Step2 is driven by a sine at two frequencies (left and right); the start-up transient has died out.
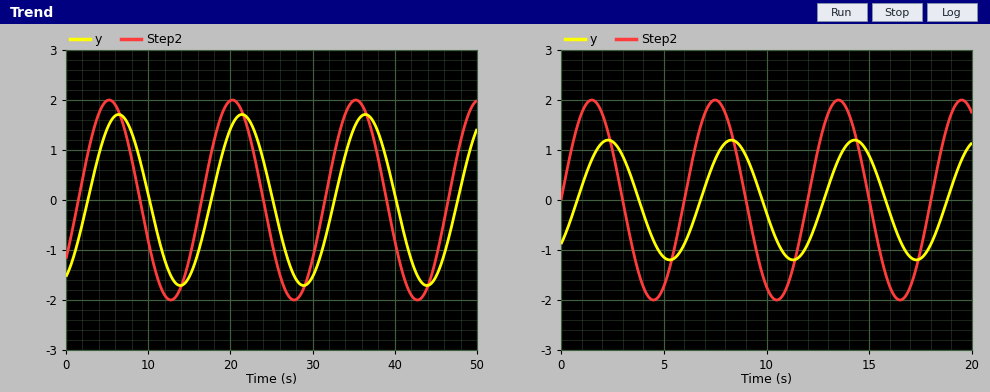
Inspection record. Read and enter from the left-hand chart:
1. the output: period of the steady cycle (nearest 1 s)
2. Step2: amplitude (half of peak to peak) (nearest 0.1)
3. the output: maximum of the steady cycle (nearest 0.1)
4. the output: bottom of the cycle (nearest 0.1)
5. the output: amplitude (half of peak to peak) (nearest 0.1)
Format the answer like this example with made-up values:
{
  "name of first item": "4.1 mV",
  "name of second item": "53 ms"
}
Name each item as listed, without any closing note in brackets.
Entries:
{
  "the output: period of the steady cycle": "15 s",
  "Step2: amplitude (half of peak to peak)": "2.0",
  "the output: maximum of the steady cycle": "1.7",
  "the output: bottom of the cycle": "-1.7",
  "the output: amplitude (half of peak to peak)": "1.7"
}
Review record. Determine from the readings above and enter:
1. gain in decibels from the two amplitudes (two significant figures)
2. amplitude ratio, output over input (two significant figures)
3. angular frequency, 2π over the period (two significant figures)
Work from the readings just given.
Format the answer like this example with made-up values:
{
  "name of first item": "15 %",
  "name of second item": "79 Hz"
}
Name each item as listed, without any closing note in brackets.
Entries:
{
  "gain in decibels from the two amplitudes": "-1.4 dB",
  "amplitude ratio, output over input": "0.85",
  "angular frequency, 2π over the period": "0.42 rad/s"
}
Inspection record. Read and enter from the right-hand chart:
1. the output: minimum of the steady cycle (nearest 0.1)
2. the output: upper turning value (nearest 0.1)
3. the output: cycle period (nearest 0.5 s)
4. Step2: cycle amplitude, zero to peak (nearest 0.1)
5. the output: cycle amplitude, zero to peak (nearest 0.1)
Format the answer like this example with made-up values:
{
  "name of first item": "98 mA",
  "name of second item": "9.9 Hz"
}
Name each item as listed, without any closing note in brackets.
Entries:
{
  "the output: minimum of the steady cycle": "-1.2",
  "the output: upper turning value": "1.2",
  "the output: cycle period": "6.0 s",
  "Step2: cycle amplitude, zero to peak": "2.0",
  "the output: cycle amplitude, zero to peak": "1.2"
}
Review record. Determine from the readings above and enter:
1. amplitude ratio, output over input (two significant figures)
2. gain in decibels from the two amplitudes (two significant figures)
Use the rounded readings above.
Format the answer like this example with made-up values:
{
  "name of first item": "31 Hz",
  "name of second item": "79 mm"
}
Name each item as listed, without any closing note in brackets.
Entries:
{
  "amplitude ratio, output over input": "0.60",
  "gain in decibels from the two amplitudes": "-4.4 dB"
}
